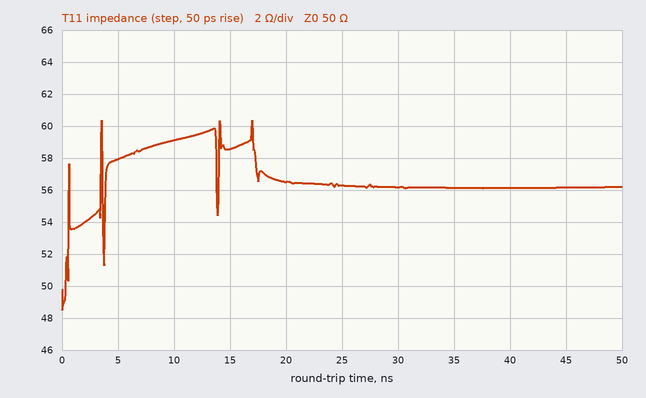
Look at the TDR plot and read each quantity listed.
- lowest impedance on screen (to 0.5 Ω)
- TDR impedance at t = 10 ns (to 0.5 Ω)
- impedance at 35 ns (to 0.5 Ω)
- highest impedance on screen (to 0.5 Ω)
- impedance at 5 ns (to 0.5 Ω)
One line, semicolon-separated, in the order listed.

48.5 Ω; 59.0 Ω; 56.0 Ω; 60.5 Ω; 58.0 Ω
